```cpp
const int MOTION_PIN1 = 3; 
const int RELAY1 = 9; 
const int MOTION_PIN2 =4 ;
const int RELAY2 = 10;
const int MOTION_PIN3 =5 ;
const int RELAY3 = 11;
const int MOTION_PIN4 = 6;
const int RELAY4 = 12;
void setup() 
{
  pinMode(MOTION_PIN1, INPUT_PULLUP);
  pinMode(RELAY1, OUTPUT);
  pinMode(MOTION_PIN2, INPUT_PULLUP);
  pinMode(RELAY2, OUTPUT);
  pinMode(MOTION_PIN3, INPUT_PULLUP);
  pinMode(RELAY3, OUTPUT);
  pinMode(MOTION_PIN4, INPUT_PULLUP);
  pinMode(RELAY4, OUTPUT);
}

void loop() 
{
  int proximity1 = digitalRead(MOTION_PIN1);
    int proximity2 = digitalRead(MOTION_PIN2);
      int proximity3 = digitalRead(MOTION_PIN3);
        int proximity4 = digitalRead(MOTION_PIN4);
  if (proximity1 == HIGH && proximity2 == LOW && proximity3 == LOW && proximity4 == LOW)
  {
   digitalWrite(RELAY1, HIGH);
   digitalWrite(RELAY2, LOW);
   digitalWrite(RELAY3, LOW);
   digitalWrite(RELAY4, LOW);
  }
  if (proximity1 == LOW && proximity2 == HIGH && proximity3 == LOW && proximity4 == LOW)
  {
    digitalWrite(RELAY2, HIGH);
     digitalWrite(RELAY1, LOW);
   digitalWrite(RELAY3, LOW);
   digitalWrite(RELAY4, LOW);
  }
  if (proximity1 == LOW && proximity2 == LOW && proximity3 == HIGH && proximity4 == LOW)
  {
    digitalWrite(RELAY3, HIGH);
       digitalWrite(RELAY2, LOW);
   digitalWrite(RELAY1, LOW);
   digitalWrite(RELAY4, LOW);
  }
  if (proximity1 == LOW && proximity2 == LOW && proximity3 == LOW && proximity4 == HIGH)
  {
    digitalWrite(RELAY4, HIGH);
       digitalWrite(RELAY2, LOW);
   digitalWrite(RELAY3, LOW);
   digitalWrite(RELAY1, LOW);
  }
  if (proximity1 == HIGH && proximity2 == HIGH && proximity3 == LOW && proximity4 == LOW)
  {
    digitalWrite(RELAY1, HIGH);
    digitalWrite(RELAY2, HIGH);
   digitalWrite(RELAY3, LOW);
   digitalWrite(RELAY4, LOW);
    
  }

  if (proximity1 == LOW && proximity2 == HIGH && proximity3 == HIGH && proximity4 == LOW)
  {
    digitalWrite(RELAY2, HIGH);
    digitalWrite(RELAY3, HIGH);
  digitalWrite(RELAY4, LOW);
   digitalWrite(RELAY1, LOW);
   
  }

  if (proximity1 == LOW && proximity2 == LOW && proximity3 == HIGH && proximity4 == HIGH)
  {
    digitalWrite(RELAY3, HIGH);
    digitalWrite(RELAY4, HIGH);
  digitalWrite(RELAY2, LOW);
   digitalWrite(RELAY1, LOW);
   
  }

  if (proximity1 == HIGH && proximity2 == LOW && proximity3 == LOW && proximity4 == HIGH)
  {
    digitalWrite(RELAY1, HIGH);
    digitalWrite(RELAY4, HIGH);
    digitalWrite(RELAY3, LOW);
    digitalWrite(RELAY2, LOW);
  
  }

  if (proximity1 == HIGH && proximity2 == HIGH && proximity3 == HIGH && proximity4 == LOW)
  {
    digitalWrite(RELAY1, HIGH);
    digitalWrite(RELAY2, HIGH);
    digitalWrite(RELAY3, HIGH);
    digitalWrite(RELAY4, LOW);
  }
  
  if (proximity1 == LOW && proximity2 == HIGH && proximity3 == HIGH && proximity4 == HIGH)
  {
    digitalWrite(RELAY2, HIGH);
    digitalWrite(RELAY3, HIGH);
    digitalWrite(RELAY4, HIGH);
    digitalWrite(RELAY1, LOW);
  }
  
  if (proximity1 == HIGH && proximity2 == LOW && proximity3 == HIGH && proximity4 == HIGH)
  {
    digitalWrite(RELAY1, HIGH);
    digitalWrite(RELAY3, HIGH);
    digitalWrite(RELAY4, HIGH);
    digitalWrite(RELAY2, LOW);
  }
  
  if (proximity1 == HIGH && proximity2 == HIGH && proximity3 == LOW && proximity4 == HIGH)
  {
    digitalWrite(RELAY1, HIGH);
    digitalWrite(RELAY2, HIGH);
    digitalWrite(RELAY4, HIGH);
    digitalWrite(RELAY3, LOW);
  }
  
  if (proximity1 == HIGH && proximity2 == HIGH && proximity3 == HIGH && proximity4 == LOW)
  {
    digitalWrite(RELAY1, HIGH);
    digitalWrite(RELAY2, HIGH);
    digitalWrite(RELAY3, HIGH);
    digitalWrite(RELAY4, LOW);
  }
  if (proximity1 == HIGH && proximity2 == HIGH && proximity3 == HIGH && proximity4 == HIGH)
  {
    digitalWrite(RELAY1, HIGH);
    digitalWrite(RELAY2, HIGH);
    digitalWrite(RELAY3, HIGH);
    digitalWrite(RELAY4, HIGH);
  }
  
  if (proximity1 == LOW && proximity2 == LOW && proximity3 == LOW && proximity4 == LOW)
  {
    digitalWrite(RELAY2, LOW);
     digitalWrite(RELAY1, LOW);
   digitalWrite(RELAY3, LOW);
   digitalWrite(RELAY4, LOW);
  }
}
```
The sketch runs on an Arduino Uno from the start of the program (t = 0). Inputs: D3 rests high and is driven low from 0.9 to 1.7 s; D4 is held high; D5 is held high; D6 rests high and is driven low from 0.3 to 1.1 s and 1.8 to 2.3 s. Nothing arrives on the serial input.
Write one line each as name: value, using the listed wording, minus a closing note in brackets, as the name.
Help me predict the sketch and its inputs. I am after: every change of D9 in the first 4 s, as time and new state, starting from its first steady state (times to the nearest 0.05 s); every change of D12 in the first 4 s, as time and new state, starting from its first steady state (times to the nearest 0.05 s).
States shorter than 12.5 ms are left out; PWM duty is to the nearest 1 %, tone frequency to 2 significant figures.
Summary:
every change of D9 in the first 4 s, as time and new state, starting from its first steady state: 0 s high; 0.9 s low; 1.7 s high
every change of D12 in the first 4 s, as time and new state, starting from its first steady state: 0 s high; 0.3 s low; 1.1 s high; 1.8 s low; 2.3 s high
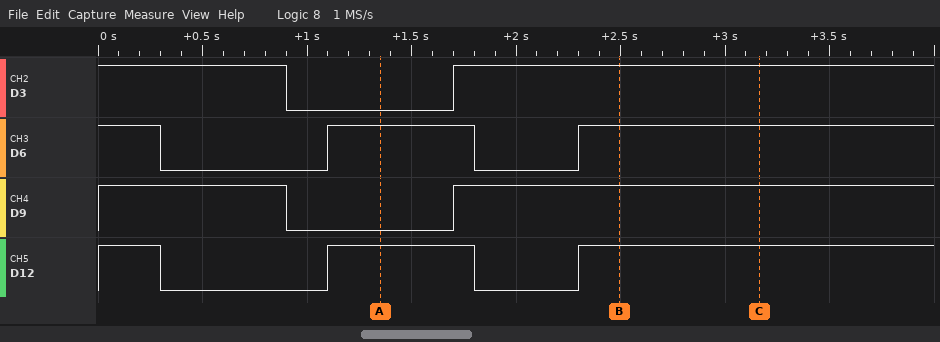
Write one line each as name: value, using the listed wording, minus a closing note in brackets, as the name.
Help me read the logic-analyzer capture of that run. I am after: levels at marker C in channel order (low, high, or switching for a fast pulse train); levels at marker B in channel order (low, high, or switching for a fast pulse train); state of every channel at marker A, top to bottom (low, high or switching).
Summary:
levels at marker C in channel order: D3 high, D6 high, D9 high, D12 high
levels at marker B in channel order: D3 high, D6 high, D9 high, D12 high
state of every channel at marker A, top to bottom: D3 low, D6 high, D9 low, D12 high
